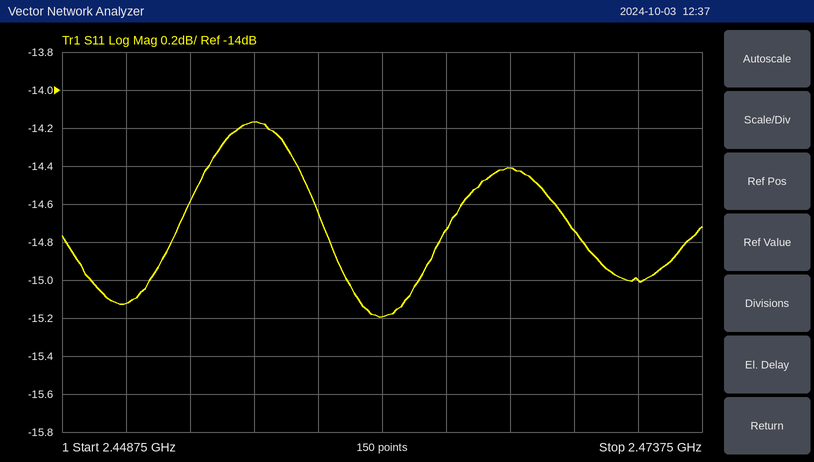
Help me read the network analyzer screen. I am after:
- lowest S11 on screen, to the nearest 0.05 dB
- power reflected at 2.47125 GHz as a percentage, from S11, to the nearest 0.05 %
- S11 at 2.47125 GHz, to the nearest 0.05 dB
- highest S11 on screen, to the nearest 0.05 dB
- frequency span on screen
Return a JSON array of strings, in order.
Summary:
["-15.20 dB", "3.15 %", "-15.00 dB", "-14.15 dB", "25 MHz"]
